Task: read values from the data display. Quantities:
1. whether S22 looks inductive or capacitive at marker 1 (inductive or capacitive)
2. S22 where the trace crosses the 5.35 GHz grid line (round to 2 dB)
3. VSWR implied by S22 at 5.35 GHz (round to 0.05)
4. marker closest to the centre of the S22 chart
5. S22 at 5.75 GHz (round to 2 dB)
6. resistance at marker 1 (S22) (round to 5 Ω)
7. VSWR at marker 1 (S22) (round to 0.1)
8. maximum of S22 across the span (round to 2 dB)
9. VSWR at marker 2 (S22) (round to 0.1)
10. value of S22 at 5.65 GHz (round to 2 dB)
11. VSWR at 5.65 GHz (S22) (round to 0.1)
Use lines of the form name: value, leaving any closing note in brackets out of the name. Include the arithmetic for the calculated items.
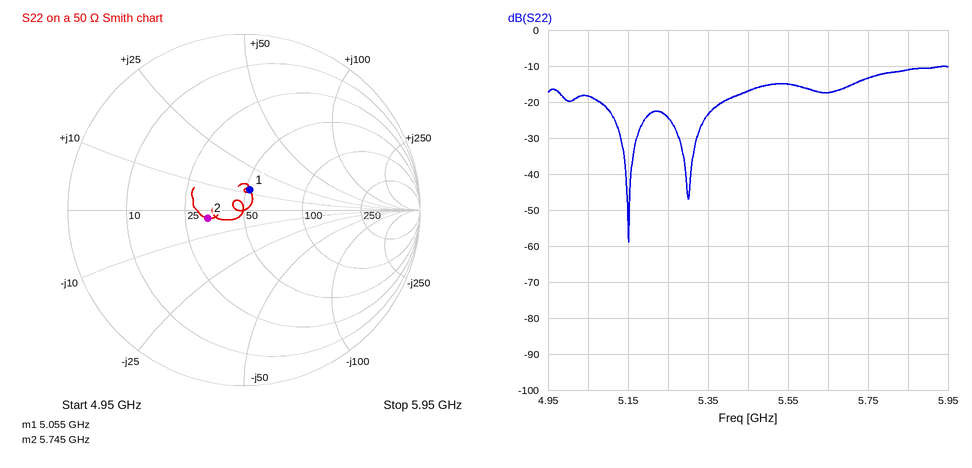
whether S22 looks inductive or capacitive at marker 1: inductive
S22 where the trace crosses the 5.35 GHz grid line: -24 dB
VSWR implied by S22 at 5.35 GHz: |Γ| = 10^(-24/20) = 0.0631; VSWR = (1 + 0.0631)/(1 − 0.0631) ≈ 1.13, so 1.15 to the nearest 0.05
marker closest to the centre of the S22 chart: marker 1
S22 at 5.75 GHz: -14 dB
resistance at marker 1 (S22): 50 Ω
VSWR at marker 1 (S22): 1.3
maximum of S22 across the span: -10 dB
VSWR at marker 2 (S22): 1.5
value of S22 at 5.65 GHz: -18 dB
VSWR at 5.65 GHz (S22): |Γ| = 10^(-18/20) = 0.1259; VSWR = (1 + 0.1259)/(1 − 0.1259) ≈ 1.3
